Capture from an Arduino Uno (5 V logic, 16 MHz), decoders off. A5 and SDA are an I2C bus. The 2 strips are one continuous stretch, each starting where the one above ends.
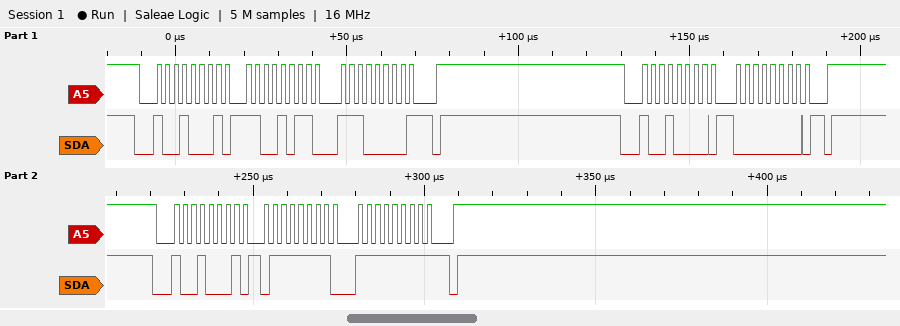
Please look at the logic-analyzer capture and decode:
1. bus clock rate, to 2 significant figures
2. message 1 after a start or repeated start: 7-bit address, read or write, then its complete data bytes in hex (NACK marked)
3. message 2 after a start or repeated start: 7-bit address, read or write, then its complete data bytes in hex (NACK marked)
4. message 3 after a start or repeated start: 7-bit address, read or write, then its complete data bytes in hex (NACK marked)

400 kHz
0x48 read: CB E0 NACK
0x48 write: 00
0x48 read: 7F FF NACK
